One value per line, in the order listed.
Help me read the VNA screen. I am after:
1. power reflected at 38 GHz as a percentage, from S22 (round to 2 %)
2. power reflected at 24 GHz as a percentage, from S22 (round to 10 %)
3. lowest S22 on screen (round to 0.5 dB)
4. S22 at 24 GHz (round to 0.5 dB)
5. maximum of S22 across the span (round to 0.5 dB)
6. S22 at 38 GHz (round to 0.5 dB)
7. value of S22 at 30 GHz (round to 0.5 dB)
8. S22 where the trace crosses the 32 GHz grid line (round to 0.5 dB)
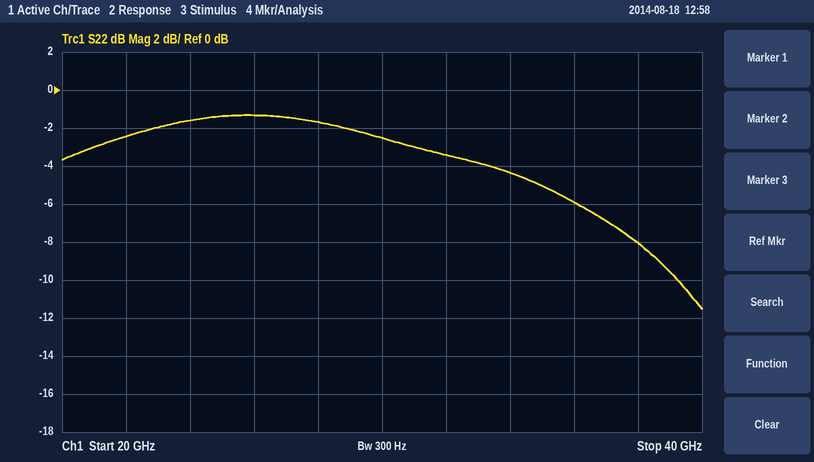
16 %
70 %
-11.5 dB
-1.5 dB
-1.5 dB
-8.0 dB
-2.5 dB
-3.5 dB
